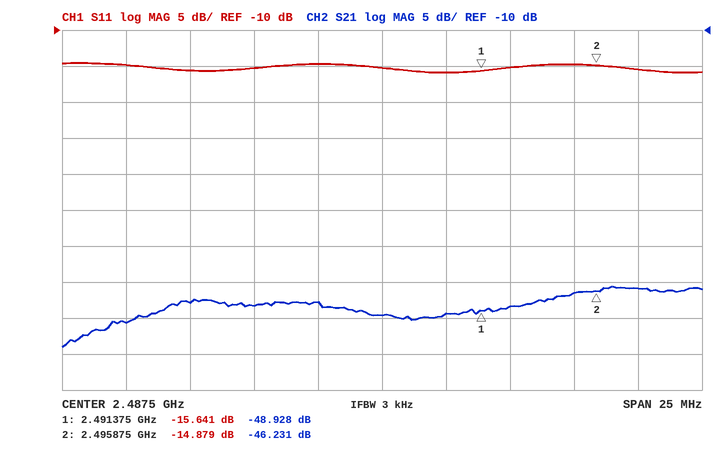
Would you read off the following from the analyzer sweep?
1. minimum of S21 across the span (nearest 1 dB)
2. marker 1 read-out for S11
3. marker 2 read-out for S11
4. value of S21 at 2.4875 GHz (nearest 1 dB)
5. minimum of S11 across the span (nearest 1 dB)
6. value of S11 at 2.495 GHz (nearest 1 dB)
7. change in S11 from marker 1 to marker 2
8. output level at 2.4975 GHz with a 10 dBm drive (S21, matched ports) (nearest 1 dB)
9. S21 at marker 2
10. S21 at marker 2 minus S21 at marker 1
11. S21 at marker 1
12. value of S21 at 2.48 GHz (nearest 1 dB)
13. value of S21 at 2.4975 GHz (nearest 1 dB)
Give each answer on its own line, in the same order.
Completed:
-54 dB
-15.641 dB
-14.879 dB
-50 dB
-16 dB
-15 dB
0.762 dB
-36 dBm
-46.231 dB
2.697 dB
-48.928 dB
-48 dB
-46 dB
